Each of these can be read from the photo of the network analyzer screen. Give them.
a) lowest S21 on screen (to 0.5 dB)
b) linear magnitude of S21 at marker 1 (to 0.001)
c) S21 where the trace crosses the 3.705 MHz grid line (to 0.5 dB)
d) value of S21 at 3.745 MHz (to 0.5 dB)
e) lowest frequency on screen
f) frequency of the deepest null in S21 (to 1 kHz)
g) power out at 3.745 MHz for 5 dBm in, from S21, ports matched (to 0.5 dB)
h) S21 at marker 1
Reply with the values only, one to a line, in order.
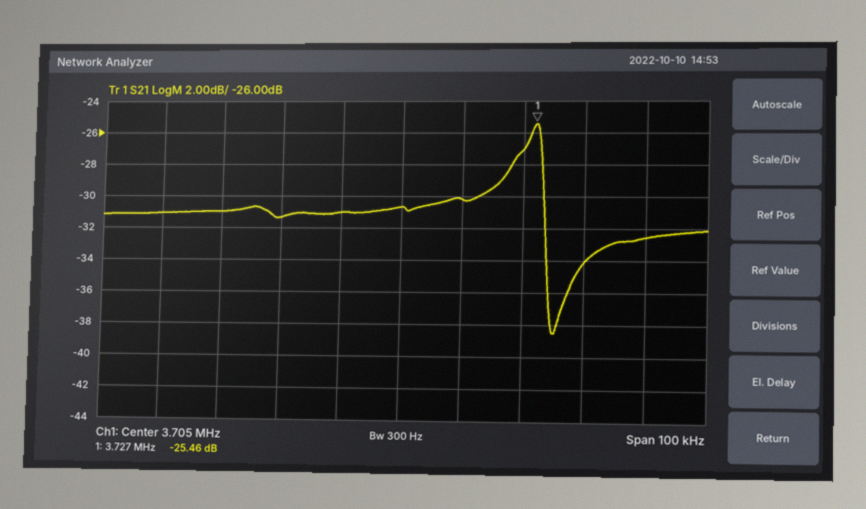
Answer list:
-38.5 dB
0.053
-30.5 dB
-32.5 dB
3.655 MHz
3.730 MHz
-27.5 dBm
-25.46 dB
